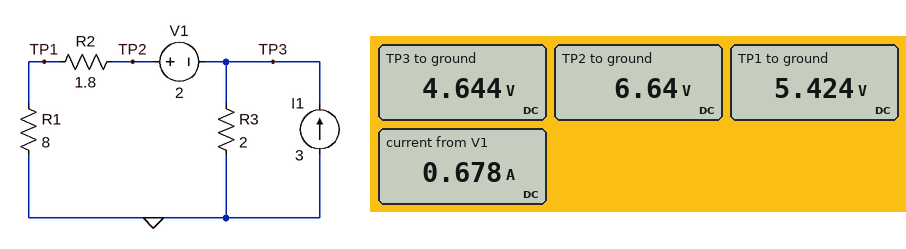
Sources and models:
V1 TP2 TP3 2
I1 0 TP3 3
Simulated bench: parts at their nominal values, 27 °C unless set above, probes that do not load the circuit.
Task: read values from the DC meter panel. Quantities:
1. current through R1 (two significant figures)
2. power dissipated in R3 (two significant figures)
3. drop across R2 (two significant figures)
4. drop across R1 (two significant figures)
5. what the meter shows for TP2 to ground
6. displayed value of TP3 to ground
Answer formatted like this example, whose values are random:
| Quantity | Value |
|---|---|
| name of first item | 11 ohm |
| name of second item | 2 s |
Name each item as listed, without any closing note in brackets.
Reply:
| Quantity | Value |
|---|---|
| current through R1 | 680 mA |
| power dissipated in R3 | 11 W |
| drop across R2 | 1.2 V |
| drop across R1 | 5.4 V |
| what the meter shows for TP2 to ground | 6.64 V |
| displayed value of TP3 to ground | 4.644 V |
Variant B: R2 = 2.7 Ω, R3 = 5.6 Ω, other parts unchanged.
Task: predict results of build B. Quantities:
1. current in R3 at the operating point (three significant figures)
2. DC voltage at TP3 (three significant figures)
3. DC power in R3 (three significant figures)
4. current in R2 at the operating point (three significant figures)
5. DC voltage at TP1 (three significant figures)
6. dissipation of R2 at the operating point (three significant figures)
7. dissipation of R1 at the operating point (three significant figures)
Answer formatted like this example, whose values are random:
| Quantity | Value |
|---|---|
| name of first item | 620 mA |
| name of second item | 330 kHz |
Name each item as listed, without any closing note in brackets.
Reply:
| Quantity | Value |
|---|---|
| current in R3 at the operating point | 1.85 A |
| DC voltage at TP3 | 10.3 V |
| DC power in R3 | 19.1 W |
| current in R2 at the operating point | 1.15 A |
| DC voltage at TP1 | 9.23 V |
| dissipation of R2 at the operating point | 3.59 W |
| dissipation of R1 at the operating point | 10.6 W |
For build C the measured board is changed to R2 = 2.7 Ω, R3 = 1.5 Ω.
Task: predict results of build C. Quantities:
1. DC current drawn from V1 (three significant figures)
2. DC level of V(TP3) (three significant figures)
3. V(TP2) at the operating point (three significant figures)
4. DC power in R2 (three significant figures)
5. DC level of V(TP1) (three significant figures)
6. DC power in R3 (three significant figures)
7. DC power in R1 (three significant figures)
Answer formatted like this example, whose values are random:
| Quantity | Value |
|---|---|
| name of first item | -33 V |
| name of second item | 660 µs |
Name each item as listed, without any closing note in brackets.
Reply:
| Quantity | Value |
|---|---|
| DC current drawn from V1 | 533 mA |
| DC level of V(TP3) | 3.70 V |
| V(TP2) at the operating point | 5.70 V |
| DC power in R2 | 766 mW |
| DC level of V(TP1) | 4.26 V |
| DC power in R3 | 9.13 W |
| DC power in R1 | 2.27 W |
